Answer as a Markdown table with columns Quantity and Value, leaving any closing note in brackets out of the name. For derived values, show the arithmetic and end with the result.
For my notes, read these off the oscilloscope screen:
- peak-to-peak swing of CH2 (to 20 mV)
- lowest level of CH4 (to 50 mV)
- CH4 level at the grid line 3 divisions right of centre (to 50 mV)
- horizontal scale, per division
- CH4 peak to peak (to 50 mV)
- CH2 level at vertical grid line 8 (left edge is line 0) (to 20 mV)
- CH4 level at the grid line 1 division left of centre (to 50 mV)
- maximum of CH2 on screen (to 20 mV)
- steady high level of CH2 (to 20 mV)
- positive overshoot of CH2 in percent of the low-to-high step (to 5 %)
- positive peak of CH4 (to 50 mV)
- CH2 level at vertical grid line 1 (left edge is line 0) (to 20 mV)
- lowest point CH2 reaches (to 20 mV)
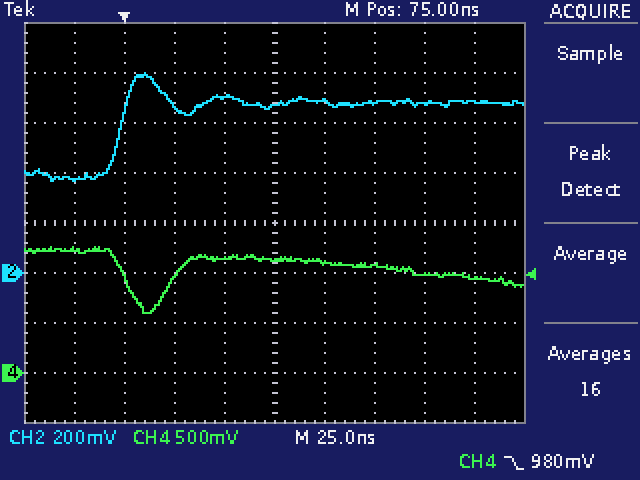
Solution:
| Quantity | Value |
|---|---|
| peak-to-peak swing of CH2 | 800 mV − (360 mV) = 440 mV |
| lowest level of CH4 | 600 mV |
| CH4 level at the grid line 3 divisions right of centre | 1.00 V |
| horizontal scale, per division | 25 ns |
| CH4 peak to peak | 1.25 V − (600 mV) = 650 mV |
| CH2 level at vertical grid line 8 (left edge is line 0) | 680 mV |
| CH4 level at the grid line 1 division left of centre | 1.15 V |
| maximum of CH2 on screen | 800 mV |
| steady high level of CH2 | 680 mV |
| positive overshoot of CH2 in percent of the low-to-high step | 40 % |
| positive peak of CH4 | 1.25 V |
| CH2 level at vertical grid line 1 (left edge is line 0) | 380 mV |
| lowest point CH2 reaches | 360 mV |
